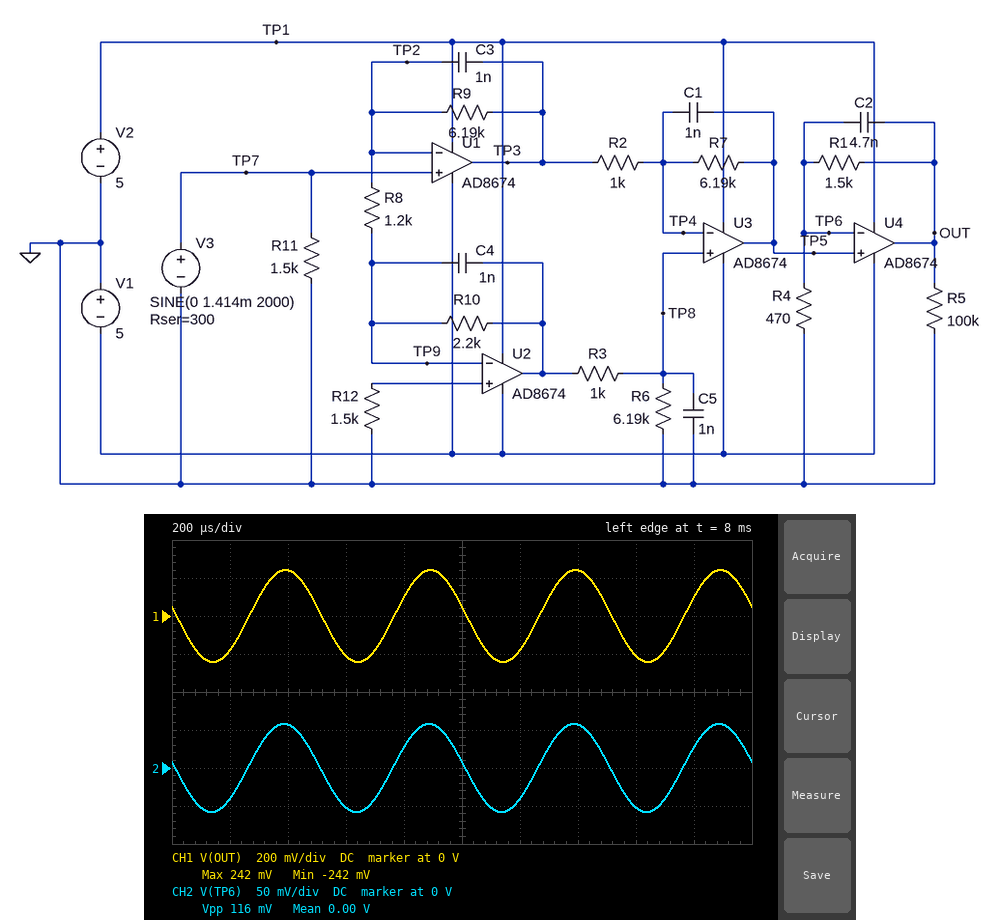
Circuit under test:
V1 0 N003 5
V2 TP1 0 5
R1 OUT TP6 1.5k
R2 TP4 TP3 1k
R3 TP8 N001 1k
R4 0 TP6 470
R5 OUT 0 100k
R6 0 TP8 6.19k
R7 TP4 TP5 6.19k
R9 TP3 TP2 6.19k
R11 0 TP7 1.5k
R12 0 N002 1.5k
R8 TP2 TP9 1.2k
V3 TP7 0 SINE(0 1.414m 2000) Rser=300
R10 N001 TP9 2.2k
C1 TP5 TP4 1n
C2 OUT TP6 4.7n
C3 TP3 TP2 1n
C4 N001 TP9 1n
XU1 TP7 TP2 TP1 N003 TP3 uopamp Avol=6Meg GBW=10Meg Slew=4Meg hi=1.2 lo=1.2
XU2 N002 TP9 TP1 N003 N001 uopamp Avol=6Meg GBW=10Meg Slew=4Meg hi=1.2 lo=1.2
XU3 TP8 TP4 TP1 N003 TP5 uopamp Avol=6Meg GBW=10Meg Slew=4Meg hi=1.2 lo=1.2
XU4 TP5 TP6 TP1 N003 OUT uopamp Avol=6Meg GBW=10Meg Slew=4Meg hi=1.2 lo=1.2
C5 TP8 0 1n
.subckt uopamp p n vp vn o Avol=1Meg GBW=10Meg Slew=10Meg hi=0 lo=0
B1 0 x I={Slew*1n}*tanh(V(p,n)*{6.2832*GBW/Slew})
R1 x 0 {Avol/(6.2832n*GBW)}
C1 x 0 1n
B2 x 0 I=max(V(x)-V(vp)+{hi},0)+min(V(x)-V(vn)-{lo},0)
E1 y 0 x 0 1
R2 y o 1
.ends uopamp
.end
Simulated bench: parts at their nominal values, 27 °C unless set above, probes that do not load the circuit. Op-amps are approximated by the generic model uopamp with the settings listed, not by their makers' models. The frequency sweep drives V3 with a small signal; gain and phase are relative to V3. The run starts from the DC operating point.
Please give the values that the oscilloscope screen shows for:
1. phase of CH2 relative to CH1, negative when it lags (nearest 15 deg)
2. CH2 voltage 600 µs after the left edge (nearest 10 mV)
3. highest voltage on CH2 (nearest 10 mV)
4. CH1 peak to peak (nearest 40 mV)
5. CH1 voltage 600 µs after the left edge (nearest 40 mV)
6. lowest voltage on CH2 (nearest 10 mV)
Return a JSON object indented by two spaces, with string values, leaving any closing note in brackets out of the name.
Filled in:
{
  "phase of CH2 relative to CH1, negative when it lags": "0 deg",
  "CH2 voltage 600 µs after the left edge": "-50 mV",
  "highest voltage on CH2": "60 mV",
  "CH1 peak to peak": "480 mV",
  "CH1 voltage 600 µs after the left edge": "-200 mV",
  "lowest voltage on CH2": "-60 mV"
}
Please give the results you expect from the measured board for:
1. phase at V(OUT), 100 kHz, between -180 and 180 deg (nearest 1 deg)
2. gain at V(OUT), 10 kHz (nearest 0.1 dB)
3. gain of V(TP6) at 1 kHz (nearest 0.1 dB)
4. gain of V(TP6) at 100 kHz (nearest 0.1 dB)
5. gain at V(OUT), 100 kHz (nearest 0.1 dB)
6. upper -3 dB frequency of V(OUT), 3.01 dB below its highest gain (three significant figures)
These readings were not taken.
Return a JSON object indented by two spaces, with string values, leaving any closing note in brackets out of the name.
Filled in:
{
  "phase at V(OUT), 100 kHz, between -180 and 180 deg": "24 deg",
  "gain at V(OUT), 10 kHz": "42.9 dB",
  "gain of V(TP6) at 1 kHz": "32.3 dB",
  "gain of V(TP6) at 100 kHz": "11.0 dB",
  "gain at V(OUT), 100 kHz": "13.5 dB",
  "upper -3 dB frequency of V(OUT), 3.01 dB below its highest gain": "13.0 kHz"
}
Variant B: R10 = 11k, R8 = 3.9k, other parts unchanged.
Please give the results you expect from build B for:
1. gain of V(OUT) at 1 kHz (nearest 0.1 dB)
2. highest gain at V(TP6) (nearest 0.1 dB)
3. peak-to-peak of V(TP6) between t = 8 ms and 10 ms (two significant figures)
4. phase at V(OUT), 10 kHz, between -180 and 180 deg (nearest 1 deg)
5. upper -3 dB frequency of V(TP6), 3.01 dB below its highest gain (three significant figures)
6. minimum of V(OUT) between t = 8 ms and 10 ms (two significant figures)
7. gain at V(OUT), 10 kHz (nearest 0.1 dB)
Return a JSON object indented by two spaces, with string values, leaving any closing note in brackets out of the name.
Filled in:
{
  "gain of V(OUT) at 1 kHz": "41.3 dB",
  "highest gain at V(TP6)": "28.9 dB",
  "peak-to-peak of V(TP6) between t = 8 ms and 10 ms": "78 mV",
  "phase at V(OUT), 10 kHz, between -180 and 180 deg": "117 deg",
  "upper -3 dB frequency of V(TP6), 3.01 dB below its highest gain": "13.1 kHz",
  "minimum of V(OUT) between t = 8 ms and 10 ms": "-160 mV",
  "gain at V(OUT), 10 kHz": "38.7 dB"
}
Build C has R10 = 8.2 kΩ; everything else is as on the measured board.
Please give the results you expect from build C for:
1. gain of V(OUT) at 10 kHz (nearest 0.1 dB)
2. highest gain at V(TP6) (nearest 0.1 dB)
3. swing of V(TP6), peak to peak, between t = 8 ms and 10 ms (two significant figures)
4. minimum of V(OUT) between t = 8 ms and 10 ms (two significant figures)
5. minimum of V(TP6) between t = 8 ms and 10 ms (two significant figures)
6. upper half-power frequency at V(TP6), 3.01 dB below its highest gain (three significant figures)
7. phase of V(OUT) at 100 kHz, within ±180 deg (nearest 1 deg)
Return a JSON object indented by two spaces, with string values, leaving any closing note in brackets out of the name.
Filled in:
{
  "gain of V(OUT) at 10 kHz": "46.7 dB",
  "highest gain at V(TP6)": "36.5 dB",
  "swing of V(TP6), peak to peak, between t = 8 ms and 10 ms": "190 mV",
  "minimum of V(OUT) between t = 8 ms and 10 ms": "-390 mV",
  "minimum of V(TP6) between t = 8 ms and 10 ms": "-94 mV",
  "upper half-power frequency at V(TP6), 3.01 dB below its highest gain": "14.7 kHz",
  "phase of V(OUT) at 100 kHz, within ±180 deg": "13 deg"
}
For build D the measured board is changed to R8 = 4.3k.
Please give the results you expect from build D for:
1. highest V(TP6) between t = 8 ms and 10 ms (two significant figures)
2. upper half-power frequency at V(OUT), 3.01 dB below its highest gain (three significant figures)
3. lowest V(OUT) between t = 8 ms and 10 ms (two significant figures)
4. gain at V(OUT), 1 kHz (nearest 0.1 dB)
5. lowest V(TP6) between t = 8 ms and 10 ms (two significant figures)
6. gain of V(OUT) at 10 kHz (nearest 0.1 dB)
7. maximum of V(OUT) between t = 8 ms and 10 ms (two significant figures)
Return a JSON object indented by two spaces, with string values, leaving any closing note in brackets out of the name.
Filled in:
{
  "highest V(TP6) between t = 8 ms and 10 ms": "21 mV",
  "upper half-power frequency at V(OUT), 3.01 dB below its highest gain": "13.3 kHz",
  "lowest V(OUT) between t = 8 ms and 10 ms": "-89 mV",
  "gain at V(OUT), 1 kHz": "36.1 dB",
  "lowest V(TP6) between t = 8 ms and 10 ms": "-21 mV",
  "gain of V(OUT) at 10 kHz": "34.3 dB",
  "maximum of V(OUT) between t = 8 ms and 10 ms": "89 mV"
}
